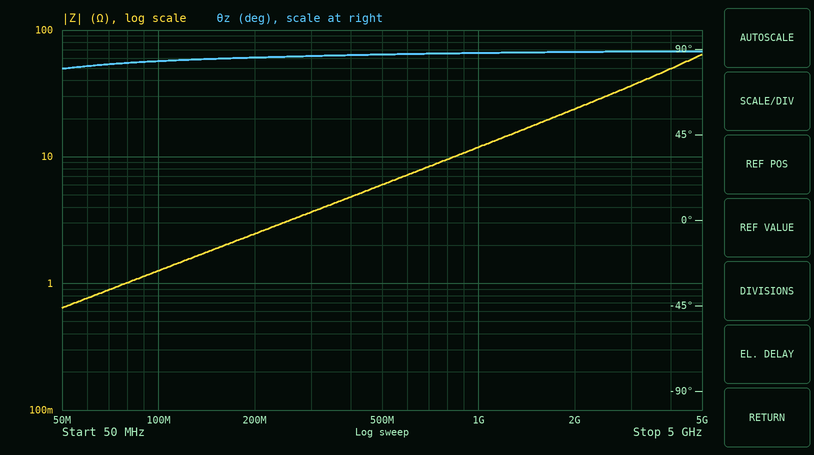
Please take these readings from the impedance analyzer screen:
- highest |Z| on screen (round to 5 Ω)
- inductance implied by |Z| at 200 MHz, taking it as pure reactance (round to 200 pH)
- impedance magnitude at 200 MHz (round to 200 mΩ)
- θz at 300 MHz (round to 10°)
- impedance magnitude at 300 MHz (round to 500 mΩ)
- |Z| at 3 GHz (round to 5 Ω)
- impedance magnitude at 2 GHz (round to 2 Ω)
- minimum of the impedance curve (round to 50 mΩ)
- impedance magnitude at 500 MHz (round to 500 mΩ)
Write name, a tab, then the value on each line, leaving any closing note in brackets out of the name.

highest |Z| on screen	65 Ω
inductance implied by |Z| at 200 MHz, taking it as pure reactance	2.0 nH
impedance magnitude at 200 MHz	2.4 Ω
θz at 300 MHz	90°
impedance magnitude at 300 MHz	3.5 Ω
|Z| at 3 GHz	35 Ω
impedance magnitude at 2 GHz	24 Ω
minimum of the impedance curve	650 mΩ
impedance magnitude at 500 MHz	6.0 Ω
